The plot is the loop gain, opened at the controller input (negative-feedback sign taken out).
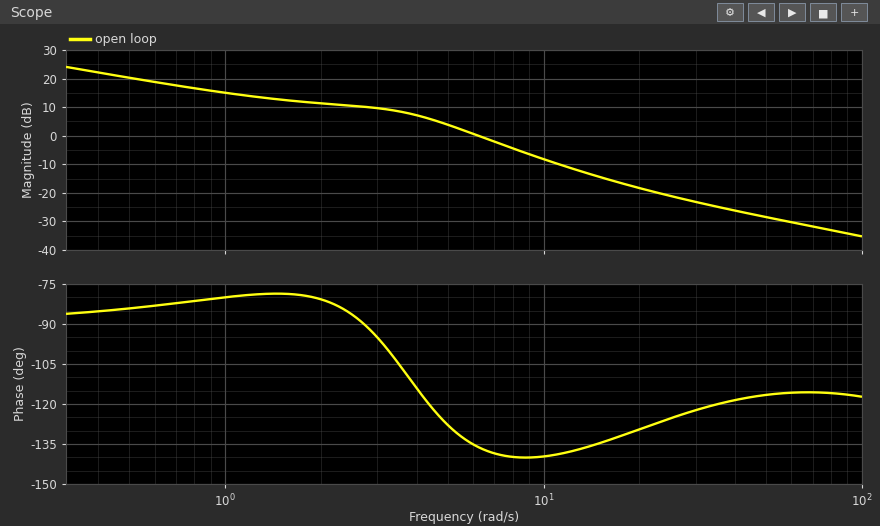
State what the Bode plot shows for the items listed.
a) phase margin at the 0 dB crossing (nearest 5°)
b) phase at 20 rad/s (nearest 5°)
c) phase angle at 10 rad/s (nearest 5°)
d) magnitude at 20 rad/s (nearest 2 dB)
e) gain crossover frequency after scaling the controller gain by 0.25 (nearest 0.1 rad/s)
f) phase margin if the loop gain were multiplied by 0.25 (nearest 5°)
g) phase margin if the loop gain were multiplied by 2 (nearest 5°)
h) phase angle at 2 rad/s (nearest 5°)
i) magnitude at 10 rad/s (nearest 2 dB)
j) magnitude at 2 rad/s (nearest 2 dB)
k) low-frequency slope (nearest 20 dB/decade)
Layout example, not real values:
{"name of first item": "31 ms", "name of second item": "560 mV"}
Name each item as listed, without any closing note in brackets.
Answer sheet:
{"phase margin at the 0 dB crossing": "45°", "phase at 20 rad/s": "-130°", "phase angle at 10 rad/s": "-140°", "magnitude at 20 rad/s": "-18 dB", "gain crossover frequency after scaling the controller gain by 0.25": "1.7 rad/s", "phase margin if the loop gain were multiplied by 0.25": "100°", "phase margin if the loop gain were multiplied by 2": "40°", "phase angle at 2 rad/s": "-80°", "magnitude at 10 rad/s": "-8 dB", "magnitude at 2 rad/s": "12 dB", "low-frequency slope": "-20 dB/decade"}
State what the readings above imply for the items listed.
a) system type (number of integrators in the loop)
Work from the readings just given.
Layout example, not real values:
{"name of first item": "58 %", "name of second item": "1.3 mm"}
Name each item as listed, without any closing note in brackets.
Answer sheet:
{"system type": "1"}
